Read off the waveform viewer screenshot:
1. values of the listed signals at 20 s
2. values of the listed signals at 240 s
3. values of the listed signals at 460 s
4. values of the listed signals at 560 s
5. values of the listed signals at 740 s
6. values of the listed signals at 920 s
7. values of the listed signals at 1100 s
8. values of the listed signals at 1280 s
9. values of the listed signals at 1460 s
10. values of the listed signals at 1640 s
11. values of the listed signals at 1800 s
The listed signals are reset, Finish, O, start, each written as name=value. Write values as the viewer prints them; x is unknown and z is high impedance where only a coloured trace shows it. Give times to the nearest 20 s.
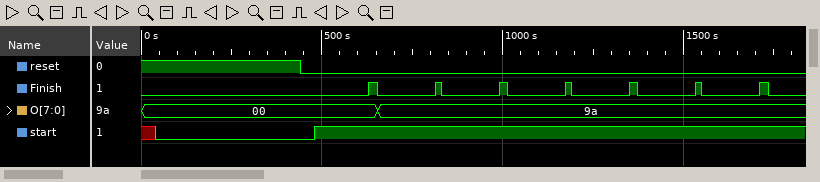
reset=1, Finish=0, O=00, start=x
reset=1, Finish=0, O=00, start=0
reset=0, Finish=0, O=00, start=0
reset=0, Finish=0, O=00, start=1
reset=0, Finish=0, O=9a, start=1
reset=0, Finish=0, O=9a, start=1
reset=0, Finish=0, O=9a, start=1
reset=0, Finish=0, O=9a, start=1
reset=0, Finish=0, O=9a, start=1
reset=0, Finish=0, O=9a, start=1
reset=0, Finish=0, O=9a, start=1
